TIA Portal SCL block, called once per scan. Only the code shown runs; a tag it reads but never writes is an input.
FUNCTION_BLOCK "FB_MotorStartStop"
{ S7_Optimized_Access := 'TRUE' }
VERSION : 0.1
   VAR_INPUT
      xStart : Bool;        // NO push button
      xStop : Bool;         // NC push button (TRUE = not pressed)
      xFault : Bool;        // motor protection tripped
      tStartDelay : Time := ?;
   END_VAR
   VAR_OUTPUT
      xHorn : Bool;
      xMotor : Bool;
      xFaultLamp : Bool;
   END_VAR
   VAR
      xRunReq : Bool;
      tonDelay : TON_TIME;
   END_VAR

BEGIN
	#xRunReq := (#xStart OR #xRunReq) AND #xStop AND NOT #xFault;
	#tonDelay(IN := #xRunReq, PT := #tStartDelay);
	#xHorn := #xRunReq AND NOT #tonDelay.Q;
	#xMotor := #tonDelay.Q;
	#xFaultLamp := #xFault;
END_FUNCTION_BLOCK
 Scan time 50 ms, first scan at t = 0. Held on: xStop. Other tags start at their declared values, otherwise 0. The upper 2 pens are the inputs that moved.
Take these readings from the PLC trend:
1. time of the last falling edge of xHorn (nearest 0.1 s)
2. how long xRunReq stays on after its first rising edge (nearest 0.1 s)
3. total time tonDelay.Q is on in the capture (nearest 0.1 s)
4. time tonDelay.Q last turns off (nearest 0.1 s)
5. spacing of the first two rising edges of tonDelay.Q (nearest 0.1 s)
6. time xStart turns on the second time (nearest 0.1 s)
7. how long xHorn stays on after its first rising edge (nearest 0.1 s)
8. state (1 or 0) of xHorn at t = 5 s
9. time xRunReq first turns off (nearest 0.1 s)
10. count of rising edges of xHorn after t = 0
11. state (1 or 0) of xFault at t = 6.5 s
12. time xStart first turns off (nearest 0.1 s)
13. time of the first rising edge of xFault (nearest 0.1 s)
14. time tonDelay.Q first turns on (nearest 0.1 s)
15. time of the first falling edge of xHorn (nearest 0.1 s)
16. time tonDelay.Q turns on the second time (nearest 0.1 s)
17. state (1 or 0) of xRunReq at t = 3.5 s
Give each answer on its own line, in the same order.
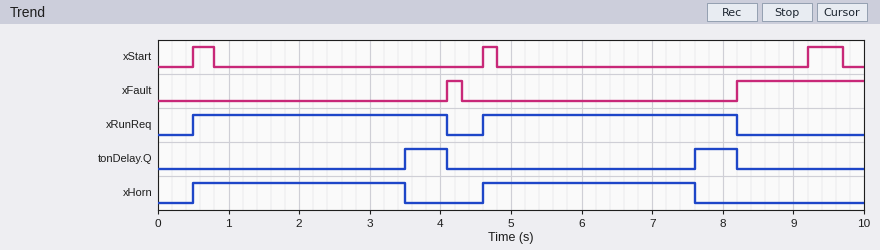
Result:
7.6 s
3.6 s
1.2 s
8.2 s
4.1 s
4.6 s
3.0 s
1
4.1 s
2
0
0.8 s
4.1 s
3.5 s
3.5 s
7.6 s
1
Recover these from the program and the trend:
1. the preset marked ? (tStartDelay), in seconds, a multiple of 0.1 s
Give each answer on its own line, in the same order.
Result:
3.0 s
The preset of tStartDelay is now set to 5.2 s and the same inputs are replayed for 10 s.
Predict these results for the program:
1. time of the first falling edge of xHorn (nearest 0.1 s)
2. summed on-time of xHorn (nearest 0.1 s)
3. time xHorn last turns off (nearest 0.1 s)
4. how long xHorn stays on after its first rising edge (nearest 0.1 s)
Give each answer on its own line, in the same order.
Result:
4.1 s
7.2 s
8.2 s
3.6 s
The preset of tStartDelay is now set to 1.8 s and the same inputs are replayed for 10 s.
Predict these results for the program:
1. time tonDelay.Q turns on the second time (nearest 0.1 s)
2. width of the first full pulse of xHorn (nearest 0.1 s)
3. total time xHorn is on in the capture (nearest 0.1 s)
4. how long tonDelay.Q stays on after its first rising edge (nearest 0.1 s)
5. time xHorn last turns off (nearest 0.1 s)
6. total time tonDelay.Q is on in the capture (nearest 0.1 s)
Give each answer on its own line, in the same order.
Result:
6.4 s
1.8 s
3.6 s
1.8 s
6.4 s
3.6 s
